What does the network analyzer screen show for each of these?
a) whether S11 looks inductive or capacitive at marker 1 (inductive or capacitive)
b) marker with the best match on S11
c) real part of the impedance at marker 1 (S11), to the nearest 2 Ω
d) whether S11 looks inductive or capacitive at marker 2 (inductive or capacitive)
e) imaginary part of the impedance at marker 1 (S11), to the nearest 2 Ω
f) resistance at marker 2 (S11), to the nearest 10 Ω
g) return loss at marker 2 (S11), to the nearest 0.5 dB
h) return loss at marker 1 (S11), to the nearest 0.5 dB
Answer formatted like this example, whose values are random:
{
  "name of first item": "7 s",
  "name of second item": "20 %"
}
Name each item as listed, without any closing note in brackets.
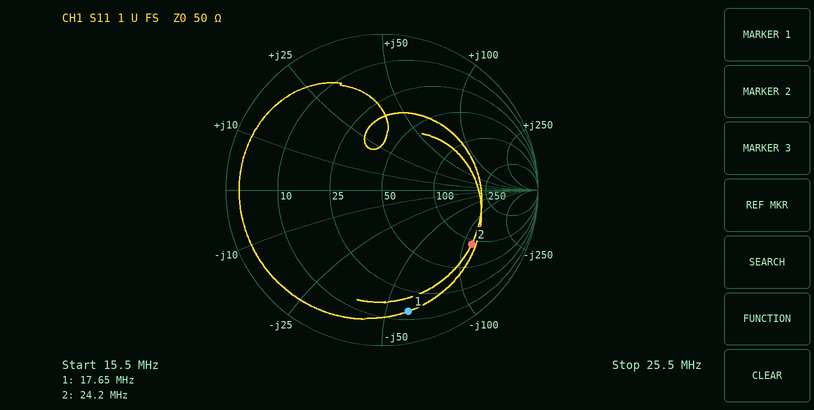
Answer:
{
  "whether S11 looks inductive or capacitive at marker 1": "capacitive",
  "marker with the best match on S11": "marker 2",
  "real part of the impedance at marker 1 (S11), to the nearest 2 Ω": "14 Ω",
  "whether S11 looks inductive or capacitive at marker 2": "capacitive",
  "imaginary part of the impedance at marker 1 (S11), to the nearest 2 Ω": "-60 Ω",
  "resistance at marker 2 (S11), to the nearest 10 Ω": "90 Ω",
  "return loss at marker 2 (S11), to the nearest 0.5 dB": "3.5 dB",
  "return loss at marker 1 (S11), to the nearest 0.5 dB": "2.0 dB"
}
